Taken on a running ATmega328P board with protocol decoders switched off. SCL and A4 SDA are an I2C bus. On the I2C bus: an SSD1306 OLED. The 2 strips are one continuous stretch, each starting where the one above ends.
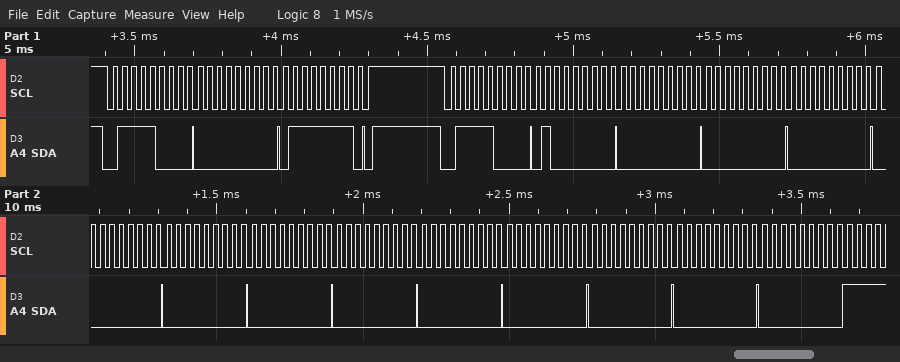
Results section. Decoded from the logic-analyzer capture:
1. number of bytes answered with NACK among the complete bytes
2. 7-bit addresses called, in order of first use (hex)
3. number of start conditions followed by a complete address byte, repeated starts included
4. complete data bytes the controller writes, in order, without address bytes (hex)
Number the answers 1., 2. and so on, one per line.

1. 0
2. 0x3C
3. 2
4. 00 7F 40 00 00 00 00 00 00 00 00 00 00 00 00
